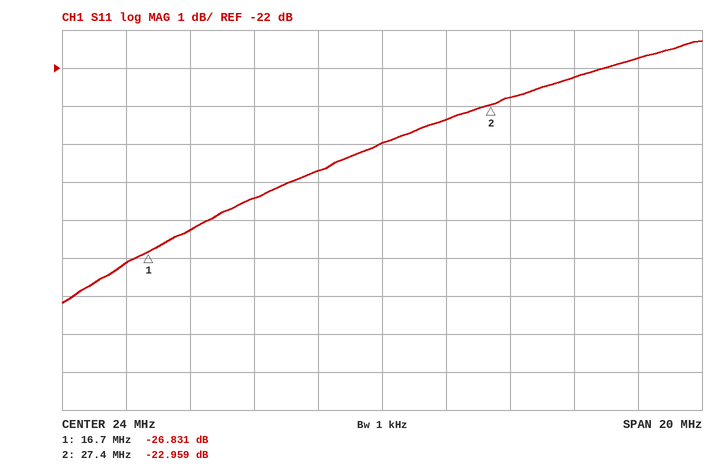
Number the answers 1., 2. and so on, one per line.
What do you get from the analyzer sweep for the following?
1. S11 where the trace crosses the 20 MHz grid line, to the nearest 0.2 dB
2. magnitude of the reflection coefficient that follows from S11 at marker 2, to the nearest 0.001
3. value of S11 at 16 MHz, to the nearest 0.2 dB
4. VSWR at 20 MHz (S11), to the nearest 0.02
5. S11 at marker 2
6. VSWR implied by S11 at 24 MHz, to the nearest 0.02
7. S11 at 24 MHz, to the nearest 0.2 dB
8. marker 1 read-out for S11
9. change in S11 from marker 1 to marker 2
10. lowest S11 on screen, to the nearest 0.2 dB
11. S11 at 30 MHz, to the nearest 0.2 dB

1. -25.4 dB
2. 0.071
3. -27.2 dB
4. 1.12
5. -22.959 dB
6. 1.14
7. -24.0 dB
8. -26.831 dB
9. 3.872 dB
10. -28.2 dB
11. -22.2 dB
